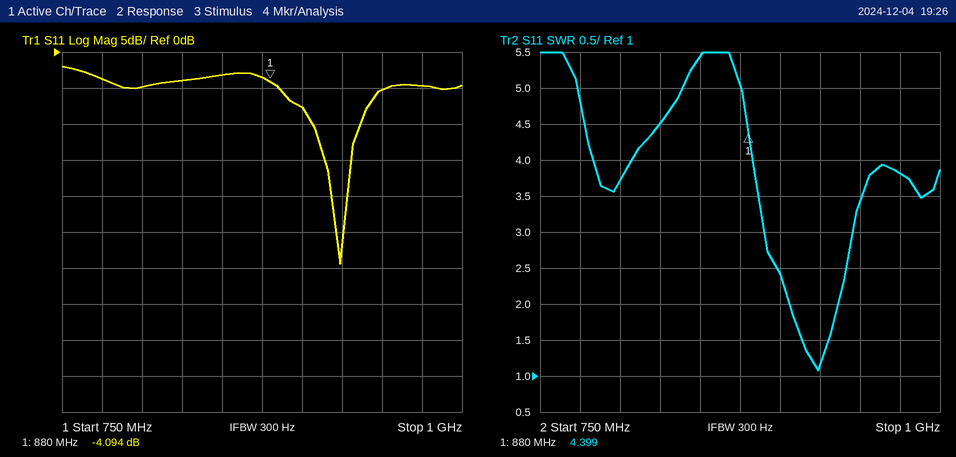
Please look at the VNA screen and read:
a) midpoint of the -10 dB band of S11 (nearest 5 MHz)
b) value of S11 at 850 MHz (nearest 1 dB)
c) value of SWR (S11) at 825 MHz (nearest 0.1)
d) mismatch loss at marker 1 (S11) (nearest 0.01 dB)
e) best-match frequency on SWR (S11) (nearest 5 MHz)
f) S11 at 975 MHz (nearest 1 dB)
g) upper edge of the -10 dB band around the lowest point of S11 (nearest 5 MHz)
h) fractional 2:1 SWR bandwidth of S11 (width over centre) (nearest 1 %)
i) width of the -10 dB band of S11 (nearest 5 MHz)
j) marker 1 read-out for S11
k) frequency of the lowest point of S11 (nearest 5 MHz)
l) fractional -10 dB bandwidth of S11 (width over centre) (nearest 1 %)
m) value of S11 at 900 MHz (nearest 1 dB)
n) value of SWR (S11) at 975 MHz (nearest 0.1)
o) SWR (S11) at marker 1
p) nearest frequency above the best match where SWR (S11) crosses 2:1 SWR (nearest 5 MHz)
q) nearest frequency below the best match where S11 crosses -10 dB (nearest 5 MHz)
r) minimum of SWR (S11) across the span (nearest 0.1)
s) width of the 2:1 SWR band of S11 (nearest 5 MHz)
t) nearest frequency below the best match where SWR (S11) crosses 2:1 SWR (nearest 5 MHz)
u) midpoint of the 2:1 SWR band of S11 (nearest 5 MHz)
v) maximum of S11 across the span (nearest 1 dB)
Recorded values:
920 MHz
-3 dB
4.5
2.14 dB
925 MHz
-5 dB
935 MHz
3 %
30 MHz
-4.094 dB
925 MHz
3 %
-8 dB
3.8
4.399
935 MHz
905 MHz
1.1
30 MHz
905 MHz
920 MHz
-2 dB
